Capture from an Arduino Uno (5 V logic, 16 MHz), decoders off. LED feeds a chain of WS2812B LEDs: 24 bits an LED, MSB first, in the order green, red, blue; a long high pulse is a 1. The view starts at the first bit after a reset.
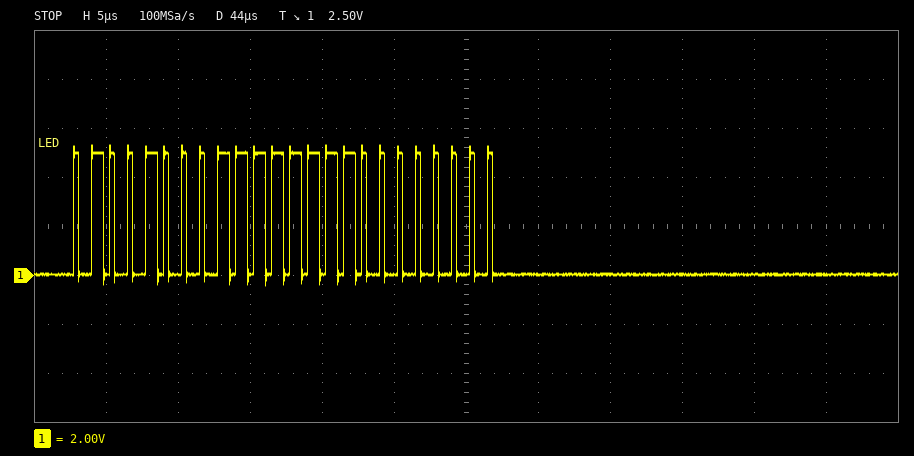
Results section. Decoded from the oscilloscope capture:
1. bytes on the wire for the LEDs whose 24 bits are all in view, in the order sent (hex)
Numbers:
48 FF 00
